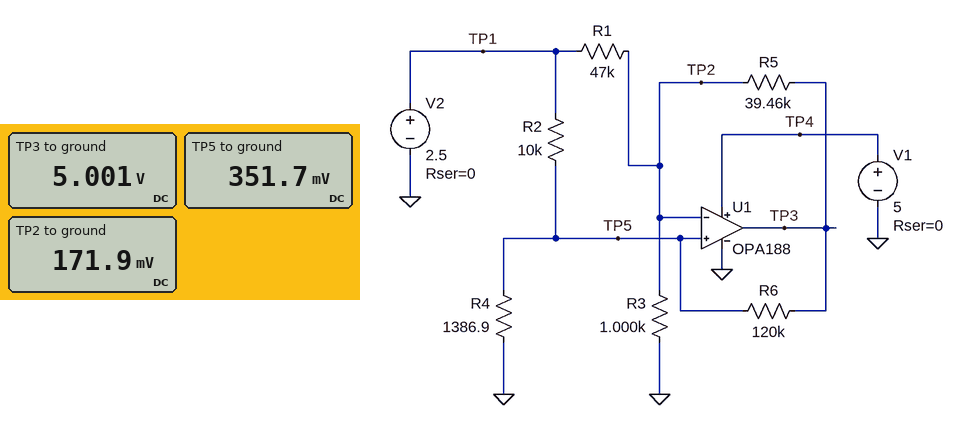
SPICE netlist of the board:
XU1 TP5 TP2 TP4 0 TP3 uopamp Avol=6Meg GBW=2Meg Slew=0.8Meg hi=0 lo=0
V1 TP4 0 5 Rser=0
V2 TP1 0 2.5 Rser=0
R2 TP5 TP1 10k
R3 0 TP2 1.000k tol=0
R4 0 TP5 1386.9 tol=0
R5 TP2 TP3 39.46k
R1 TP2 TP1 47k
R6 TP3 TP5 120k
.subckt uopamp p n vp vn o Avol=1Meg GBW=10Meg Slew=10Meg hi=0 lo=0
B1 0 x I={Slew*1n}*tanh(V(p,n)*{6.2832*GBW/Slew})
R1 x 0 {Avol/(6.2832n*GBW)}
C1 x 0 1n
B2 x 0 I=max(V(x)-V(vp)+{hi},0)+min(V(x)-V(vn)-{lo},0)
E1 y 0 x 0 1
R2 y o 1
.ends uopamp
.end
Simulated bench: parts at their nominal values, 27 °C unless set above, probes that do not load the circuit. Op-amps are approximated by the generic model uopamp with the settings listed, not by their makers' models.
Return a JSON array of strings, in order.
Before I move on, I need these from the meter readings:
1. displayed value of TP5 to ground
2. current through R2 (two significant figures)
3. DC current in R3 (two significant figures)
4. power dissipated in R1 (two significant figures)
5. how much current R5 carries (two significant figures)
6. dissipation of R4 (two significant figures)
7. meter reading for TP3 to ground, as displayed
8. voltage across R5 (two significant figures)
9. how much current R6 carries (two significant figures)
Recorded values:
["351.7 mV", "210 µA", "170 µA", "120 µW", "120 µA", "89 µW", "5.001 V", "4.8 V", "39 µA"]
